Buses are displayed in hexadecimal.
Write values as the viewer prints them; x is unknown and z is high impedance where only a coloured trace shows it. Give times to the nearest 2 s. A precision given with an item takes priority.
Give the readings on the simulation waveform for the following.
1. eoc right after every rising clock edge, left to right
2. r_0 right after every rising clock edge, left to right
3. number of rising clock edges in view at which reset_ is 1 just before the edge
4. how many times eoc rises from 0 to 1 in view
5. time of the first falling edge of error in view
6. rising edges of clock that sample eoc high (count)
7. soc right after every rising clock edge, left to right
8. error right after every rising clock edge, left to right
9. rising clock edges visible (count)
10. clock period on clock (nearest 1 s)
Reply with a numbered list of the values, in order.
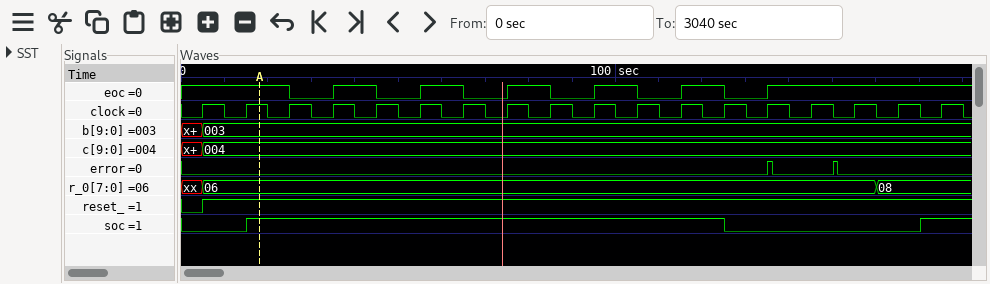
1. 1 1 0 1 0 1 0 1 0 1 0 1 0 1 1 1 1 1
2. 06, 06, 06, 06, 06, 06, 06, 06, 06, 06, 06, 06, 06, 06, 06, 06, 08, 08
3. 17
4. 6
5. 136 s
6. 12
7. 0 1 1 1 1 1 1 1 1 1 1 1 0 0 0 0 0 1
8. 0 0 0 0 0 0 0 0 0 0 0 0 0 1 0 0 0 0
9. 18
10. 10 s
